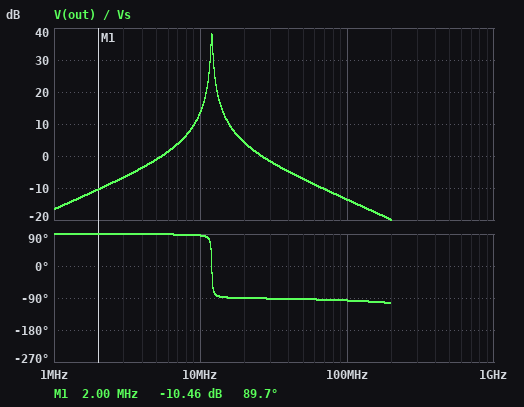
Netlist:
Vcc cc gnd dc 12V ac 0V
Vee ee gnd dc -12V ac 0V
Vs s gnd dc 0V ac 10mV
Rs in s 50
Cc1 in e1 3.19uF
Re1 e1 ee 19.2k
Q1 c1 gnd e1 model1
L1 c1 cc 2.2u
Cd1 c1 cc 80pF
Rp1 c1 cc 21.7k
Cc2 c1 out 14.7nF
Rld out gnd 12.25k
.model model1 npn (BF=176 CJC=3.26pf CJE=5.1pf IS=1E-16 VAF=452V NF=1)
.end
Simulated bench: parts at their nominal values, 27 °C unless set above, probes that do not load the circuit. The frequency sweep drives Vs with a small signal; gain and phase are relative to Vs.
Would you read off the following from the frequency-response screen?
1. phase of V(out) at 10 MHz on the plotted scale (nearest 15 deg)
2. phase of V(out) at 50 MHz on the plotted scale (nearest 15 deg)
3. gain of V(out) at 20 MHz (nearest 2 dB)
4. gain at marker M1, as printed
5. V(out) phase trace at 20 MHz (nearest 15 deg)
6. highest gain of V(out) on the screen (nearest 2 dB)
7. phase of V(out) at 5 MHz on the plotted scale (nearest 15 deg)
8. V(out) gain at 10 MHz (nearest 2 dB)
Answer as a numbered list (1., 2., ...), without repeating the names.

1. 90 deg
2. -90 deg
3. 4 dB
4. -10.46 dB
5. -90 deg
6. 38 dB
7. 90 deg
8. 14 dB
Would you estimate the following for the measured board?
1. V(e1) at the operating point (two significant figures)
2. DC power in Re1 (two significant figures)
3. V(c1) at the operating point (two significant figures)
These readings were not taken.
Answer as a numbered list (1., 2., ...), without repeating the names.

1. -760 mV
2. 6.6 mW
3. 12 V
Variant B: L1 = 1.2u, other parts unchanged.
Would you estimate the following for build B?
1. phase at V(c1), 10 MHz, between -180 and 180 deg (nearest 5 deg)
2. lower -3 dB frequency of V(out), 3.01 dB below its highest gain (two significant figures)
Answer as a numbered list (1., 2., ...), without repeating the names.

1. 90 deg
2. 16 MHz
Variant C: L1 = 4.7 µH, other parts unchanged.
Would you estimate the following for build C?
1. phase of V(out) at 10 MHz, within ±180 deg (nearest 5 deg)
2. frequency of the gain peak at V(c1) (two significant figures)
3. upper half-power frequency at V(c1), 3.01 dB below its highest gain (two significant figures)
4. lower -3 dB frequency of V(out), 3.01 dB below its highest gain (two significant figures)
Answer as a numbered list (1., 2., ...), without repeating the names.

1. -85 deg
2. 8.1 MHz
3. 8.3 MHz
4. 8.0 MHz
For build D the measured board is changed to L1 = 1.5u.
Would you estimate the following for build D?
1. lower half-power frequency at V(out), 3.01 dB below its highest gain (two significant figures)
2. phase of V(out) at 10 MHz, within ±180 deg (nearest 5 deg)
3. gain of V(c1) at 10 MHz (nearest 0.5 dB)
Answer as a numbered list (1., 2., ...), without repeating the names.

1. 14 MHz
2. 90 deg
3. 5.5 dB
